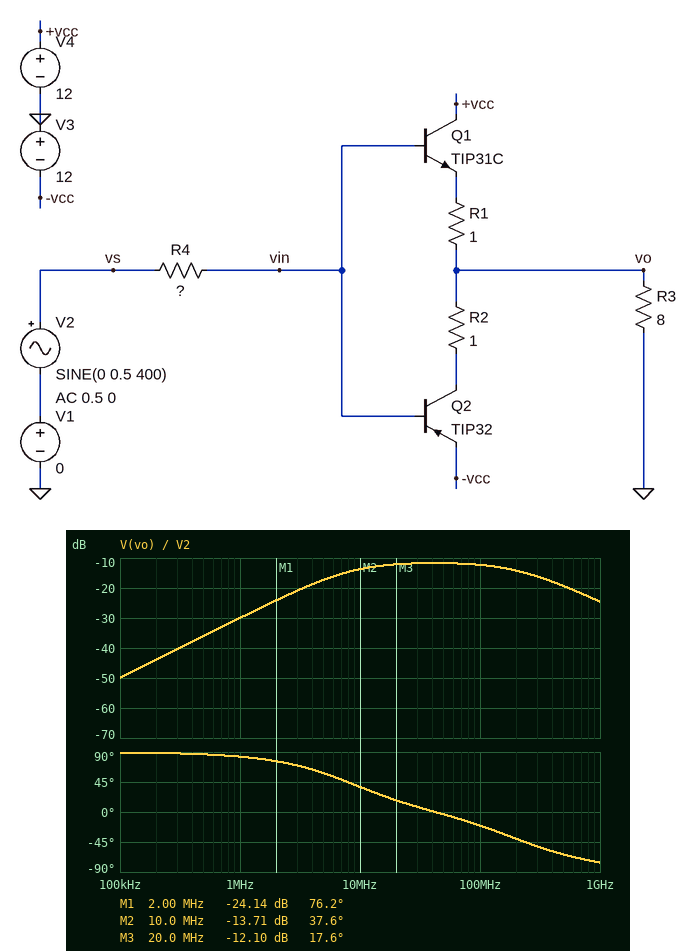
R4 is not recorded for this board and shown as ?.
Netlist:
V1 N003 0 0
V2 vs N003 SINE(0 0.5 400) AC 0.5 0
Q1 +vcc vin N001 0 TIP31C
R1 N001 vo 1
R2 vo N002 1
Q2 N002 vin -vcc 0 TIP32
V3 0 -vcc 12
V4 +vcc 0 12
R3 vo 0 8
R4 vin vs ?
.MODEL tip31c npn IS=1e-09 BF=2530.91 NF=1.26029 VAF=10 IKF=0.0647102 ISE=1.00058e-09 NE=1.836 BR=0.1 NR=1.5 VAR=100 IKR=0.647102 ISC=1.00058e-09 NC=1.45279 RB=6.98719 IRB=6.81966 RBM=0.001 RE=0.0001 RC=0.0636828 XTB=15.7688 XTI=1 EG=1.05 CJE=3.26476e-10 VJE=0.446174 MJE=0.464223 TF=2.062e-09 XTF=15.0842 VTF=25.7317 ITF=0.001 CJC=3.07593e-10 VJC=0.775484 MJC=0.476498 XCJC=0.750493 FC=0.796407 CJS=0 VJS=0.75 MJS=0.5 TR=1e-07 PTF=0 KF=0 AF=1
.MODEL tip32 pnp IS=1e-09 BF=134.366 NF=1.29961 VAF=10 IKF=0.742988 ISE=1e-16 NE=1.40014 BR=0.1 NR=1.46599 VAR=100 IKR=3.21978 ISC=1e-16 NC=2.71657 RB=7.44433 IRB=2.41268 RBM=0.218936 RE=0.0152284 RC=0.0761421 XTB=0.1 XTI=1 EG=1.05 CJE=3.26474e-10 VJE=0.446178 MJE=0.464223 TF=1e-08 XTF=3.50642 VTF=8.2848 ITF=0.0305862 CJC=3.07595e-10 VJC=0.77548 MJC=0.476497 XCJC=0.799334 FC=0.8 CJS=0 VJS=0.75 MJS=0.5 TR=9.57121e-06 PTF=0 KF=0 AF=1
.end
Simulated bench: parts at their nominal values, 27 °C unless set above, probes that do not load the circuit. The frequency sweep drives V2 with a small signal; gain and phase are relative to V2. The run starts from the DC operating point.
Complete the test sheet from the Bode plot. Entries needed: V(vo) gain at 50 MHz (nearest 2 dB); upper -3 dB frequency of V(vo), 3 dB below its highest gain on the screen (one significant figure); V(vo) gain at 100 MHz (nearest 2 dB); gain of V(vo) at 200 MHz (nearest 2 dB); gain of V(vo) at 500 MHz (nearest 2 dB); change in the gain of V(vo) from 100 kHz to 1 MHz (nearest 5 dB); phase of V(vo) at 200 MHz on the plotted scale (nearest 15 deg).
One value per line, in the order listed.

-12 dB
200 MHz
-12 dB
-14 dB
-20 dB
20 dB
-45 deg
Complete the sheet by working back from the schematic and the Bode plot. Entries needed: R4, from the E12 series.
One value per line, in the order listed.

15 Ω
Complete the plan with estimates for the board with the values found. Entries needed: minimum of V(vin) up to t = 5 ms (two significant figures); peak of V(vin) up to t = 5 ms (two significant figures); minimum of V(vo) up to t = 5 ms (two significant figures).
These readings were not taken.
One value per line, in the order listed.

-480 mV
500 mV
-13 mV
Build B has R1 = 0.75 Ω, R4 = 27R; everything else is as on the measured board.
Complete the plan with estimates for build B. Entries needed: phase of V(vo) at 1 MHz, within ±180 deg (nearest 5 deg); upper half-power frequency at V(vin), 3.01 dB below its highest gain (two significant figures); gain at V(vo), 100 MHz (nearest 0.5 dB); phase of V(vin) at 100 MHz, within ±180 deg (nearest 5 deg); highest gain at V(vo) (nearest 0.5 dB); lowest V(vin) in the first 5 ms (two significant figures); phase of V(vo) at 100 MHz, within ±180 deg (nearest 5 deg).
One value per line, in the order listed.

80 deg
6.1 MHz
-16.0 dB
-30 deg
-15.0 dB
-470 mV
-25 deg
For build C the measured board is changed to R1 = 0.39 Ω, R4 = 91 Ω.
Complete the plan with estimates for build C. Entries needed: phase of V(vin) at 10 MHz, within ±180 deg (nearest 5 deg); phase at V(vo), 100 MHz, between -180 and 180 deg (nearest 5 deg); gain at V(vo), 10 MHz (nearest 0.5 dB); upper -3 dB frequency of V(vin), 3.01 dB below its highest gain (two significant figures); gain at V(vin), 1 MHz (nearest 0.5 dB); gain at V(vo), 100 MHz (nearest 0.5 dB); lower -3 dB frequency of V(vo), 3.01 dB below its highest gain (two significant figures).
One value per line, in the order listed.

-55 deg
-30 deg
-24.0 dB
2.1 MHz
-1.0 dB
-25.0 dB
2.0 MHz
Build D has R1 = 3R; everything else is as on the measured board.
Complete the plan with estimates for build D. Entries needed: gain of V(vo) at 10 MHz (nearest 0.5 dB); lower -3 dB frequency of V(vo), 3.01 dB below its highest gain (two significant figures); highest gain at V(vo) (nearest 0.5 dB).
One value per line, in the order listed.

-14.0 dB
7.7 MHz
-12.0 dB
